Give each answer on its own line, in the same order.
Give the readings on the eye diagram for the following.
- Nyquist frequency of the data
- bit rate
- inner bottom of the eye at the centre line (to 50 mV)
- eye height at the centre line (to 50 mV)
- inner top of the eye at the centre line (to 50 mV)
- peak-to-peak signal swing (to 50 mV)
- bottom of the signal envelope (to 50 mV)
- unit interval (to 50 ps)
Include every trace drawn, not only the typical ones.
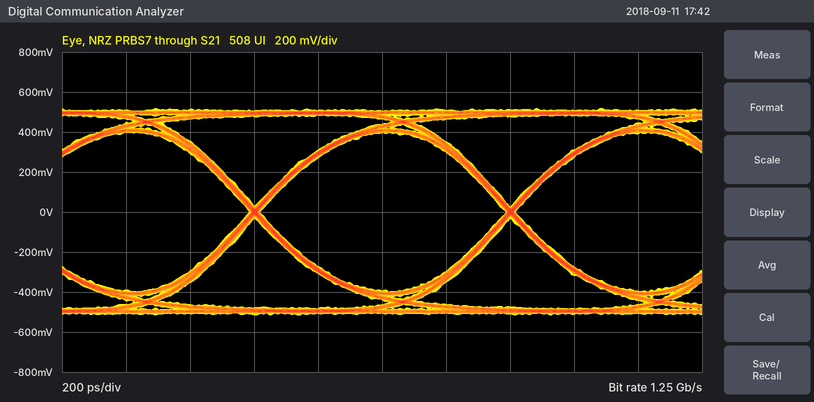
625 MHz
1.25 Gb/s
-400 mV
800 mV
400 mV
1.05 V
-500 mV
800 ps
